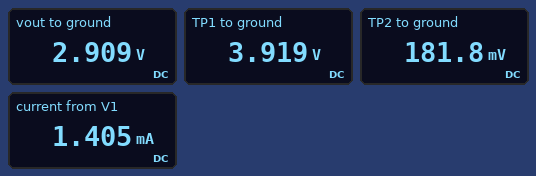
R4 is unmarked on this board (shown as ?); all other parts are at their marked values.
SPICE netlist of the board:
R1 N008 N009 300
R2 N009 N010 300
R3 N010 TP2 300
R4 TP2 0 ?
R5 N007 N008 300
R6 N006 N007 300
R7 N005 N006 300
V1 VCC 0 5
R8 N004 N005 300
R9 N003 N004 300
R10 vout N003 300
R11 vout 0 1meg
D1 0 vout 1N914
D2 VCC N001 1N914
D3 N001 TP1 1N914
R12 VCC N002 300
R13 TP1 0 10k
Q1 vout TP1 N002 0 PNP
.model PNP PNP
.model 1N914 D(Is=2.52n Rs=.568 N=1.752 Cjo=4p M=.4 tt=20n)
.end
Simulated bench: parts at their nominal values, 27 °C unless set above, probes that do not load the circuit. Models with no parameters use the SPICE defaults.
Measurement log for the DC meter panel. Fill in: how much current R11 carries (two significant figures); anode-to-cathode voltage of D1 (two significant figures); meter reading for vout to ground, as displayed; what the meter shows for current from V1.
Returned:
2.9 µA
-2.9 V
2.909 V
1.405 mA
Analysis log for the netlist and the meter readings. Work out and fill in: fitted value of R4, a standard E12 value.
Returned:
180 Ω
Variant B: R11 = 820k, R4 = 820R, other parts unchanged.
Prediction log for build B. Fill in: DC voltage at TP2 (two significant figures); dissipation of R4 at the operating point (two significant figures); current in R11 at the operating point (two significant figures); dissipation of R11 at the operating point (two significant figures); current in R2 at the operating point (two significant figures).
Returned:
830 mV
830 µW
4.3 µA
15 µW
1.0 mA
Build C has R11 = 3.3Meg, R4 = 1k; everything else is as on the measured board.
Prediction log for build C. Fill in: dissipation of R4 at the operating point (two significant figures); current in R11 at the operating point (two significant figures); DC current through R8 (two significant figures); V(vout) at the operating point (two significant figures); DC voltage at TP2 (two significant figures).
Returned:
1.0 mW
1.1 µA
1.0 mA
3.7 V
1.0 V
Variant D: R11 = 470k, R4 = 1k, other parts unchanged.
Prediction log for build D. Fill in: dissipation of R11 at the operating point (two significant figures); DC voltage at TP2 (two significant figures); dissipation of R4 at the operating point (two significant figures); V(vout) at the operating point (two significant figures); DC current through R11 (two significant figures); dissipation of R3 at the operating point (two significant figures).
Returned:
29 µW
1.0 V
1.0 mW
3.7 V
7.9 µA
300 µW
